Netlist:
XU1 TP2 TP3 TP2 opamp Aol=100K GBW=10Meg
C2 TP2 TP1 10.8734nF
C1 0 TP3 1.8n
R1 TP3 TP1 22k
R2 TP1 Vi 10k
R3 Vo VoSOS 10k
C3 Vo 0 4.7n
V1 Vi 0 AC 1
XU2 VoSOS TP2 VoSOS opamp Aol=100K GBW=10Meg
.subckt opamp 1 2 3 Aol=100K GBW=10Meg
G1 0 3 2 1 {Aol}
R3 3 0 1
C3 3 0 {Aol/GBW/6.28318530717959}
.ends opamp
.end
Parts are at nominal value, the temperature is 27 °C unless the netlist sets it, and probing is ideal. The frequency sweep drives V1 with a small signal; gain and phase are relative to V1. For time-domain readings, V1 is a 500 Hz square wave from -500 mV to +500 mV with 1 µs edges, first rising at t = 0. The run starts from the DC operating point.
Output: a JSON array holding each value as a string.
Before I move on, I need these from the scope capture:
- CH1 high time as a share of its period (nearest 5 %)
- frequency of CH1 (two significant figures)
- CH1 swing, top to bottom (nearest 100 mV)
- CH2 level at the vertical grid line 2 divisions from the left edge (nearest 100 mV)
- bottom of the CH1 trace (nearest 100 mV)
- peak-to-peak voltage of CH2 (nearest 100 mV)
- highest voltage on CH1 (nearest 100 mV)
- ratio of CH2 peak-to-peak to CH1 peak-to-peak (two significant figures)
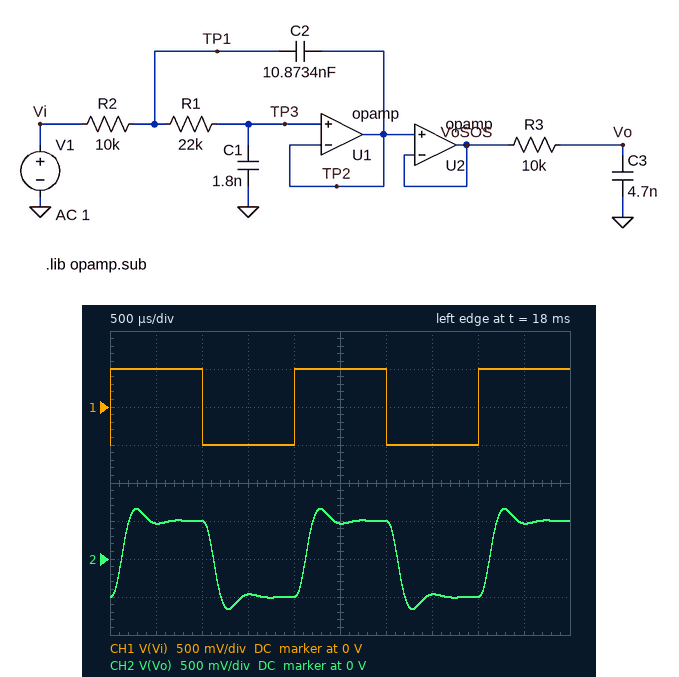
["50 %", "500 Hz", "1.0 V", "500 mV", "-500 mV", "1.3 V", "500 mV", "1.3"]
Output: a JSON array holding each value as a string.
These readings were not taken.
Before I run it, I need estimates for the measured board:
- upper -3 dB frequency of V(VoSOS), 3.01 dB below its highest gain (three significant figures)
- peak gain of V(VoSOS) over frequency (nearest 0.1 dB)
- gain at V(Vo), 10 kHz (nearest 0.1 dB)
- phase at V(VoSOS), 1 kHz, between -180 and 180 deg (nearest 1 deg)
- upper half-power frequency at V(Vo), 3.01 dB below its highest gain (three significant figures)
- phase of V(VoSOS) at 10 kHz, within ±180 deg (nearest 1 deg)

["2.87 kHz", "2.1 dB", "-34.2 dB", "-24 deg", "2.67 kHz", "-167 deg"]
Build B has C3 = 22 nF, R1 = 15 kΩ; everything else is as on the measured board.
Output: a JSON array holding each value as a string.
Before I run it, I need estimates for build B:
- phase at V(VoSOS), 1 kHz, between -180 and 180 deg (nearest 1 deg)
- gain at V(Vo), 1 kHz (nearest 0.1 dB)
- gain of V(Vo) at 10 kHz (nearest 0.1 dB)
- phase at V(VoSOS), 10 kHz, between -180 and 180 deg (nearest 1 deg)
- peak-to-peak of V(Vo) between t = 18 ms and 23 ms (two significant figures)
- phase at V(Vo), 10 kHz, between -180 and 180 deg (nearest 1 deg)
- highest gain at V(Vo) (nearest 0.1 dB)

["-18 deg", "-4.0 dB", "-43.6 dB", "-165 deg", "980 mV", "109 deg", "0 dB"]
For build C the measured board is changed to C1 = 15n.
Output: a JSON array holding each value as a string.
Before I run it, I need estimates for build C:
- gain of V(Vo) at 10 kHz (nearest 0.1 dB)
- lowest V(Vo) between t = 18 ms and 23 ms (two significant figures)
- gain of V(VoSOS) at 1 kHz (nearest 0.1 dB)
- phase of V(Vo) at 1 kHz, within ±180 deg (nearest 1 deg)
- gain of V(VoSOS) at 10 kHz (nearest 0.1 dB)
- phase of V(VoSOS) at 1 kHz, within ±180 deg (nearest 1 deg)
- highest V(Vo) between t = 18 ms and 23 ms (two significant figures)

["-53.0 dB", "-400 mV", "-9.7 dB", "-114 deg", "-43.2 dB", "-98 deg", "400 mV"]
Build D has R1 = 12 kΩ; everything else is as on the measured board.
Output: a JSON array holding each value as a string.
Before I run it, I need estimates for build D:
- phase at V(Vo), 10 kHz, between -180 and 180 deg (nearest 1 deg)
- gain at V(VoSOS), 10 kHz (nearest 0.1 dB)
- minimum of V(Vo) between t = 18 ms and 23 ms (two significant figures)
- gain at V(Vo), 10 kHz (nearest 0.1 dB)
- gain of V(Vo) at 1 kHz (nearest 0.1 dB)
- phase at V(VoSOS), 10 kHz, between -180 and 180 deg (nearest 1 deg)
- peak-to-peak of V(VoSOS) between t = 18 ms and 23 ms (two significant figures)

["125 deg", "-18.7 dB", "-640 mV", "-28.6 dB", "0.2 dB", "-163 deg", "1.5 V"]
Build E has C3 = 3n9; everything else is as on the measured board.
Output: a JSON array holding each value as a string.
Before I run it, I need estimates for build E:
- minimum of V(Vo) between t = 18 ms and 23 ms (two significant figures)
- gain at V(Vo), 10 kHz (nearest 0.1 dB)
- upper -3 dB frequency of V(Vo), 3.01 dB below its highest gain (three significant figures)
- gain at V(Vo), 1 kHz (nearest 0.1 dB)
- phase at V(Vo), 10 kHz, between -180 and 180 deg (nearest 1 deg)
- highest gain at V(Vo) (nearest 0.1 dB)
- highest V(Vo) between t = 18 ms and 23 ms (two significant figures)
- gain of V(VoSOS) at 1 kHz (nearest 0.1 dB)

["-670 mV", "-32.8 dB", "2.72 kHz", "0.6 dB", "125 deg", "1.3 dB", "670 mV", "0.9 dB"]
